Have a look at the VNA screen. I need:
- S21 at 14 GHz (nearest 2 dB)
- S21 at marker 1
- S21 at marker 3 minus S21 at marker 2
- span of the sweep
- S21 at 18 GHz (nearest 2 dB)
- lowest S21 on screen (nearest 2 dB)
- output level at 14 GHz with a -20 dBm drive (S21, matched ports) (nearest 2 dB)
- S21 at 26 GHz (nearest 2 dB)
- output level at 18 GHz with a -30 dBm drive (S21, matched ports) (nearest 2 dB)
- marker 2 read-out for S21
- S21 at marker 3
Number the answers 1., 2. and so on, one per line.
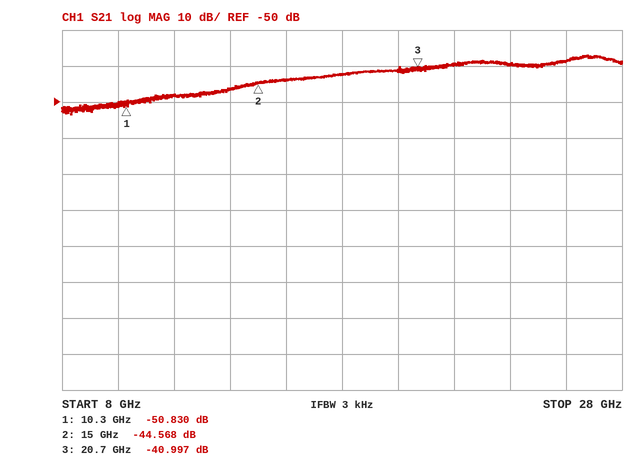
1. -46 dB
2. -50.830 dB
3. 3.571 dB
4. 20 GHz
5. -42 dB
6. -54 dB
7. -66 dBm
8. -38 dB
9. -72 dBm
10. -44.568 dB
11. -40.997 dB
